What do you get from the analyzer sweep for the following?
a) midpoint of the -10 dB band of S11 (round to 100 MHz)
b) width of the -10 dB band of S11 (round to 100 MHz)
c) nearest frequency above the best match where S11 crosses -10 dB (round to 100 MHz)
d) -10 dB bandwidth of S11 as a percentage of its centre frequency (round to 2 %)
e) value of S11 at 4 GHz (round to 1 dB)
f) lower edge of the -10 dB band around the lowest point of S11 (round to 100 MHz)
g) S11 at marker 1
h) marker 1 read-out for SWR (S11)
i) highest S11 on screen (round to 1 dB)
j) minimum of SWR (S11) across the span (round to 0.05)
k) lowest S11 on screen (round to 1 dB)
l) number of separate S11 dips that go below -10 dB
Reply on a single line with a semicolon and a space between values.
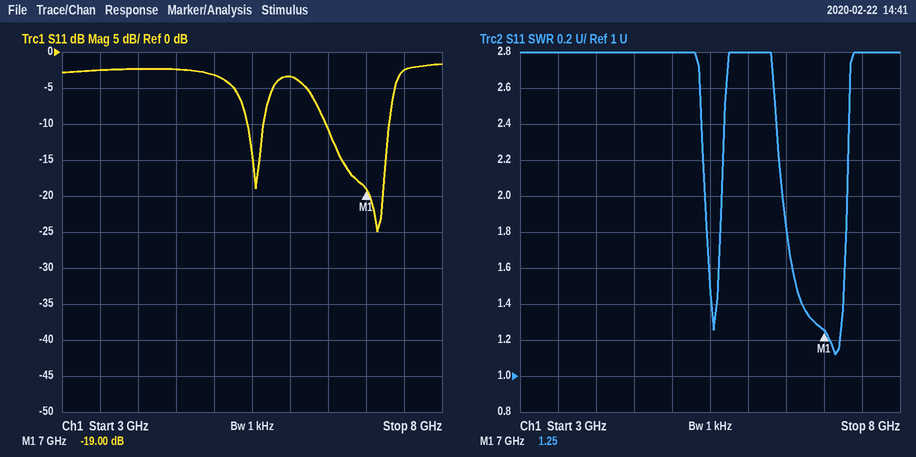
6.9 GHz; 800 MHz; 7.3 GHz; 12 %; -2 dB; 6.5 GHz; -19.00 dB; 1.25; -2 dB; 1.10; -25 dB; 2
